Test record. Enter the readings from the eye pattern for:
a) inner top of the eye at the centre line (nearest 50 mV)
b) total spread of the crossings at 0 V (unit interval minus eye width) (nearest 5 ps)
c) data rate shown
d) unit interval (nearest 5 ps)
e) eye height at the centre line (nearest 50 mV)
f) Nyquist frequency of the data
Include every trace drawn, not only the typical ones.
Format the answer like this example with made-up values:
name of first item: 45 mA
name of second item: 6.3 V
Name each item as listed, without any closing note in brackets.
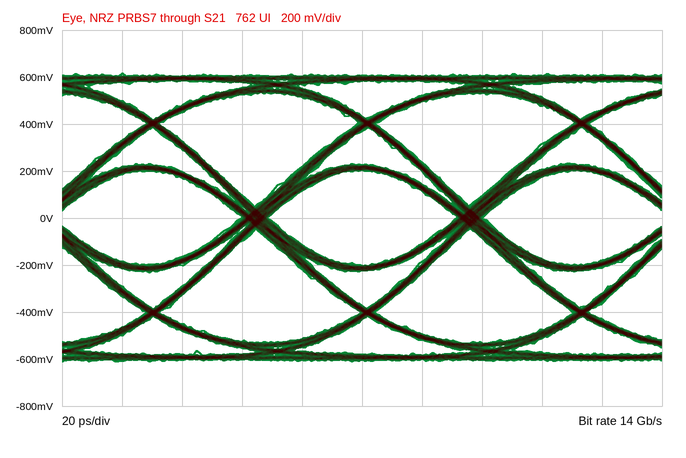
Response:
inner top of the eye at the centre line: 200 mV
total spread of the crossings at 0 V (unit interval minus eye width): 10 ps
data rate shown: 14 Gb/s
unit interval: 70 ps
eye height at the centre line: 400 mV
Nyquist frequency of the data: 7 GHz
